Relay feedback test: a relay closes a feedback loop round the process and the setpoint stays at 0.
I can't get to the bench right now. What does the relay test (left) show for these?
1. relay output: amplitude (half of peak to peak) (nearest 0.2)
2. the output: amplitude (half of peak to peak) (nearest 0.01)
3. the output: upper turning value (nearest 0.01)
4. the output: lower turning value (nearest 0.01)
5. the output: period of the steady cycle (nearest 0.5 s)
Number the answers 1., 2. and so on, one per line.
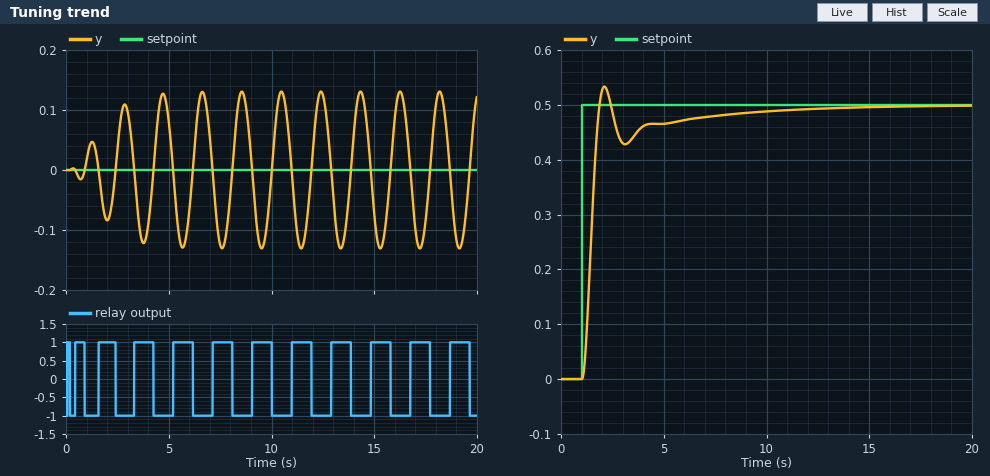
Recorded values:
1. 1.0
2. 0.13
3. 0.13
4. -0.13
5. 2.0 s
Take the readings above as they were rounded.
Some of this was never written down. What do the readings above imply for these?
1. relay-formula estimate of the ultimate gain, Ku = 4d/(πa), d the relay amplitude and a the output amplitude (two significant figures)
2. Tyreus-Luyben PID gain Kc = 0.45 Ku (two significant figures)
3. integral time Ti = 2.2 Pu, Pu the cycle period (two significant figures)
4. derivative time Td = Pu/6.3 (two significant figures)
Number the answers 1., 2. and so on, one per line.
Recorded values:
1. 9.8
2. 4.4
3. 4.4 s
4. 0.32 s
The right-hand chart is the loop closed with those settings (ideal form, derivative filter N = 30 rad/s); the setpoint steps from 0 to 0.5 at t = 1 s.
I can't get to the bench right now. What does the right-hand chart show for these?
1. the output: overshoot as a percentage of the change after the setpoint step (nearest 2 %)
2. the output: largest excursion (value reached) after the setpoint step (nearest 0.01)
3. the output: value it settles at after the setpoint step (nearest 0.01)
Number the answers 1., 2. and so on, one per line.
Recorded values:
1. 6 %
2. 0.53
3. 0.50
